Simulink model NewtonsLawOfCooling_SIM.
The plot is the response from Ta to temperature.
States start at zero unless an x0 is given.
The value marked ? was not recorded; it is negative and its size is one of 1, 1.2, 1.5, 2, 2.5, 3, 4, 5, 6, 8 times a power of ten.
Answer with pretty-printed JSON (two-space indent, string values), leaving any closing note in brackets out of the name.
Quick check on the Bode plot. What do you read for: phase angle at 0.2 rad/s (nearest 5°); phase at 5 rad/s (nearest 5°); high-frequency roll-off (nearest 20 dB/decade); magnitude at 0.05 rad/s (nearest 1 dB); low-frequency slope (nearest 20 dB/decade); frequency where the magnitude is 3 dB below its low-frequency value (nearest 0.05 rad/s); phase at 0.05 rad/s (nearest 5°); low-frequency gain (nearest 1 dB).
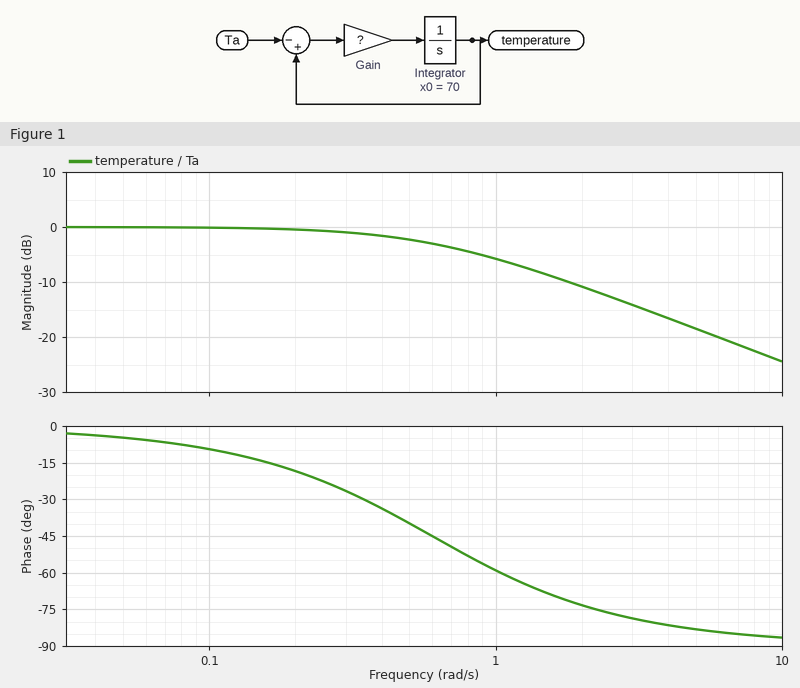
{
  "phase angle at 0.2 rad/s": "-20°",
  "phase at 5 rad/s": "-85°",
  "high-frequency roll-off": "-20 dB/decade",
  "magnitude at 0.05 rad/s": "0 dB",
  "low-frequency slope": "0 dB/decade",
  "frequency where the magnitude is 3 dB below its low-frequency value": "0.60 rad/s",
  "phase at 0.05 rad/s": "-5°",
  "low-frequency gain": "0 dB"
}
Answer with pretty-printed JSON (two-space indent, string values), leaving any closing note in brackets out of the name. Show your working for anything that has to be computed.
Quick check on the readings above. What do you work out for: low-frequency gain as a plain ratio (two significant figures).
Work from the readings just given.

{
  "low-frequency gain as a plain ratio": "10^(0 / 20) = 1.0"
}
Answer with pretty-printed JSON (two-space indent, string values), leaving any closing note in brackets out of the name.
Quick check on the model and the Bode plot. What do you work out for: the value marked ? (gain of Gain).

{
  "the value marked ?": "-0.6"
}
